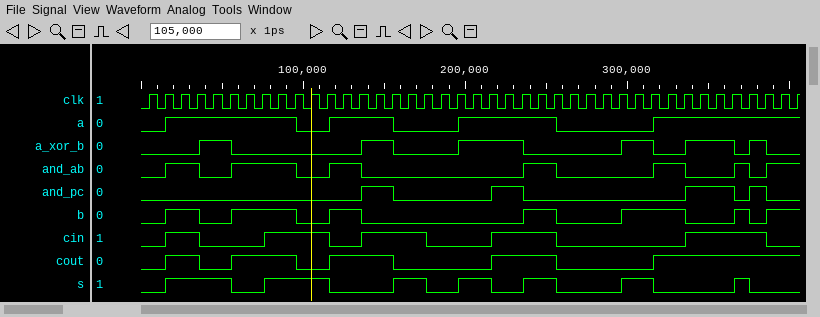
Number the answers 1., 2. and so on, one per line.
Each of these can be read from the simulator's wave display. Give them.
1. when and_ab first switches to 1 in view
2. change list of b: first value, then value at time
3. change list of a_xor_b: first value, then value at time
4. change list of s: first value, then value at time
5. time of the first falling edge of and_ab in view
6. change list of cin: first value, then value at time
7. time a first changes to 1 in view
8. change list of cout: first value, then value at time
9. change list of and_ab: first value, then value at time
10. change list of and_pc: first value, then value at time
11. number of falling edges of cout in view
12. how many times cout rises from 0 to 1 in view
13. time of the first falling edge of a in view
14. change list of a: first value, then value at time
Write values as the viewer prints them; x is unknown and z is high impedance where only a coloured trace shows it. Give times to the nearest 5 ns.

1. 15 ns
2. 0, 1 at 15 ns, 0 at 35 ns, 1 at 55 ns, 0 at 95 ns, 1 at 115 ns, 0 at 135 ns, 1 at 235 ns, 0 at 255 ns, 1 at 295 ns, 0 at 335 ns, 1 at 365 ns, 0 at 375 ns, 1 at 385 ns
3. 0, 1 at 35 ns, 0 at 55 ns, 1 at 135 ns, 0 at 155 ns, 1 at 195 ns, 0 at 235 ns, 1 at 295 ns, 0 at 315 ns, 1 at 335 ns, 0 at 365 ns, 1 at 375 ns, 0 at 385 ns
4. 0, 1 at 15 ns, 0 at 55 ns, 1 at 75 ns, 0 at 115 ns, 1 at 155 ns, 0 at 175 ns, 1 at 195 ns, 0 at 215 ns, 1 at 235 ns, 0 at 255 ns, 1 at 295 ns, 0 at 315 ns, 1 at 365 ns, 0 at 375 ns
5. 35 ns
6. 0, 1 at 15 ns, 0 at 35 ns, 1 at 75 ns, 0 at 115 ns, 1 at 135 ns, 0 at 175 ns, 1 at 215 ns, 0 at 255 ns, 1 at 335 ns, 0 at 385 ns
7. 15 ns
8. 0, 1 at 15 ns, 0 at 35 ns, 1 at 55 ns, 0 at 95 ns, 1 at 115 ns, 0 at 155 ns, 1 at 215 ns, 0 at 255 ns, 1 at 315 ns
9. 0, 1 at 15 ns, 0 at 35 ns, 1 at 55 ns, 0 at 95 ns, 1 at 115 ns, 0 at 135 ns, 1 at 235 ns, 0 at 255 ns, 1 at 315 ns, 0 at 335 ns, 1 at 365 ns, 0 at 375 ns, 1 at 385 ns
10. 0, 1 at 135 ns, 0 at 155 ns, 1 at 215 ns, 0 at 235 ns, 1 at 335 ns, 0 at 365 ns, 1 at 375 ns, 0 at 385 ns
11. 4
12. 5
13. 95 ns
14. 0, 1 at 15 ns, 0 at 95 ns, 1 at 115 ns, 0 at 155 ns, 1 at 195 ns, 0 at 255 ns, 1 at 315 ns
